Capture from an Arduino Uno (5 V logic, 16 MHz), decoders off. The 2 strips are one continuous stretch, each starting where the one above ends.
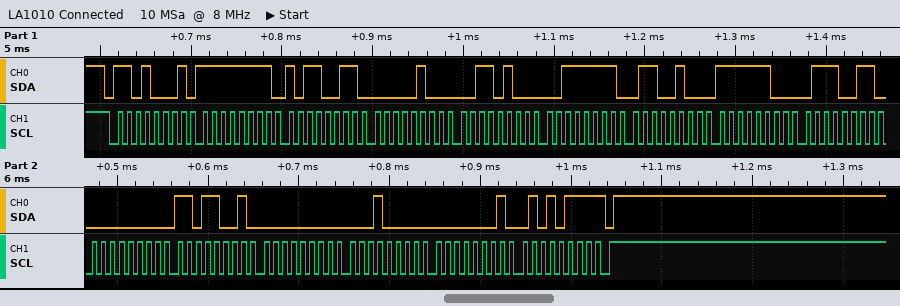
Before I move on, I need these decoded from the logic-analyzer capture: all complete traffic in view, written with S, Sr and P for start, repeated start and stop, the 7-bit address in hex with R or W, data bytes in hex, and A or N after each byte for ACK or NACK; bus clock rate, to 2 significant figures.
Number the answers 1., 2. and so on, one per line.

1. S 68R A FF A B3 A 04 A 34 A 3F A 64 A FC A 73 A 00 A D9 A 00 A 10 A 01 A 57 N P
2. 100 kHz
